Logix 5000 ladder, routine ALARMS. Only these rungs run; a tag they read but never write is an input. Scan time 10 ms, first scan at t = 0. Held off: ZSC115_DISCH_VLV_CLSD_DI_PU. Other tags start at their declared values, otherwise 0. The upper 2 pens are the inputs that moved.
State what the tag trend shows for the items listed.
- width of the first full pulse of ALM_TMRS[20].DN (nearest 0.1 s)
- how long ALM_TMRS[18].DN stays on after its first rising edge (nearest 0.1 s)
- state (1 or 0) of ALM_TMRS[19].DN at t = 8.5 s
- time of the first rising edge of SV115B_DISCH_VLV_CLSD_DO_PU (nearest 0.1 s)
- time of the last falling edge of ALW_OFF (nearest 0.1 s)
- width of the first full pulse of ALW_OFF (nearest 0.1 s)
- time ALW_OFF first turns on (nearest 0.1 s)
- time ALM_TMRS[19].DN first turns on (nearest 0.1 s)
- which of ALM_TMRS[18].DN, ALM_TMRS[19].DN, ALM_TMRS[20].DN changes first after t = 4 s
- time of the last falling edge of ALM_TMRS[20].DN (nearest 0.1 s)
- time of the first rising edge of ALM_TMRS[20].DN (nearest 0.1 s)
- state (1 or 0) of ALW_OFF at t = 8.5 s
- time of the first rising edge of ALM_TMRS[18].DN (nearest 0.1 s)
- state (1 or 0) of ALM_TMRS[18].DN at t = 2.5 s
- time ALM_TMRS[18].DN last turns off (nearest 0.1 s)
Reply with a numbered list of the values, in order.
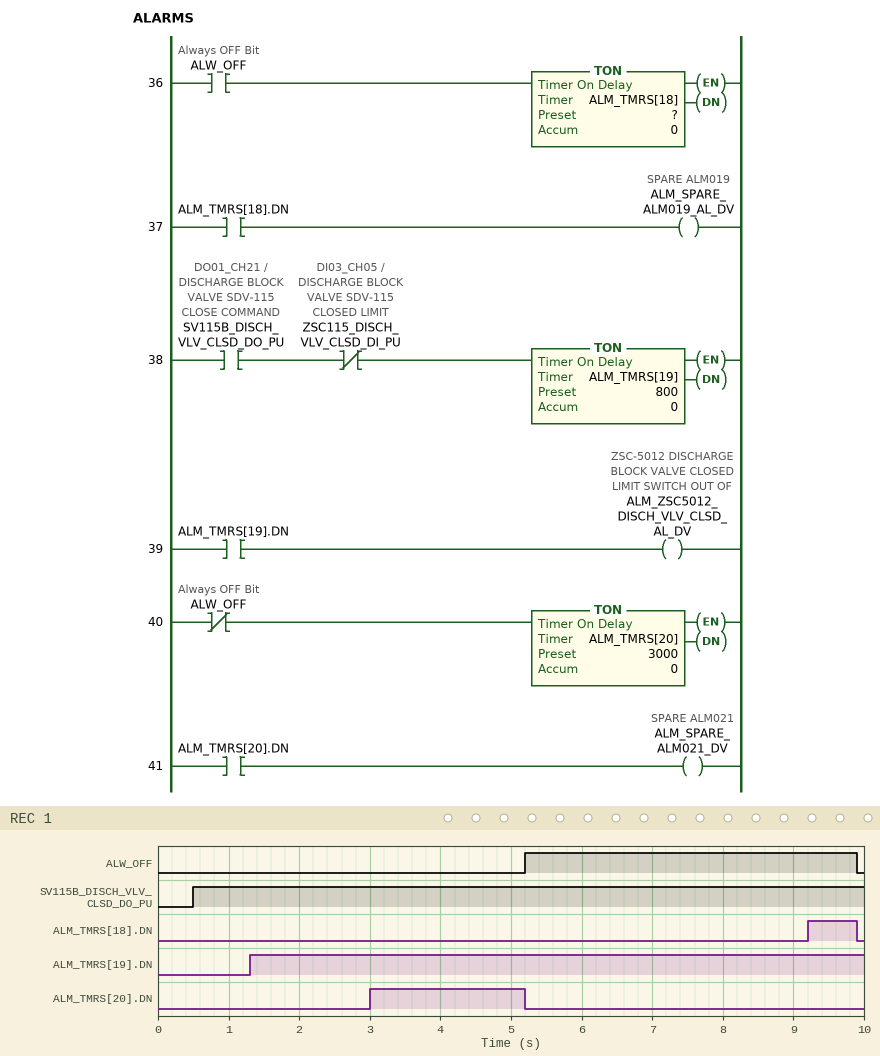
1. 2.2 s
2. 0.7 s
3. 1
4. 0.5 s
5. 9.9 s
6. 4.7 s
7. 5.2 s
8. 1.3 s
9. ALM_TMRS[20].DN
10. 5.2 s
11. 3.0 s
12. 1
13. 9.2 s
14. 0
15. 9.9 s
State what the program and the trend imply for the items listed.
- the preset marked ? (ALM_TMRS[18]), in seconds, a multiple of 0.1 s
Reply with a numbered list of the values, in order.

1. 4.0 s
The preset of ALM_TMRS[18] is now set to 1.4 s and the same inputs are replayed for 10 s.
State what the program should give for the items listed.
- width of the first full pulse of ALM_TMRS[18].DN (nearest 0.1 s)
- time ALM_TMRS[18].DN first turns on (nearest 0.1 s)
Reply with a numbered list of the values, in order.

1. 3.3 s
2. 6.6 s
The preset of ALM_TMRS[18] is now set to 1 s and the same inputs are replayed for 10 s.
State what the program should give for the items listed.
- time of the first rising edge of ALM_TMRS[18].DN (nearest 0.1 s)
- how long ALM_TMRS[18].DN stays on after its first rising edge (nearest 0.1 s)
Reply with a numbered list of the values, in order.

1. 6.2 s
2. 3.7 s
